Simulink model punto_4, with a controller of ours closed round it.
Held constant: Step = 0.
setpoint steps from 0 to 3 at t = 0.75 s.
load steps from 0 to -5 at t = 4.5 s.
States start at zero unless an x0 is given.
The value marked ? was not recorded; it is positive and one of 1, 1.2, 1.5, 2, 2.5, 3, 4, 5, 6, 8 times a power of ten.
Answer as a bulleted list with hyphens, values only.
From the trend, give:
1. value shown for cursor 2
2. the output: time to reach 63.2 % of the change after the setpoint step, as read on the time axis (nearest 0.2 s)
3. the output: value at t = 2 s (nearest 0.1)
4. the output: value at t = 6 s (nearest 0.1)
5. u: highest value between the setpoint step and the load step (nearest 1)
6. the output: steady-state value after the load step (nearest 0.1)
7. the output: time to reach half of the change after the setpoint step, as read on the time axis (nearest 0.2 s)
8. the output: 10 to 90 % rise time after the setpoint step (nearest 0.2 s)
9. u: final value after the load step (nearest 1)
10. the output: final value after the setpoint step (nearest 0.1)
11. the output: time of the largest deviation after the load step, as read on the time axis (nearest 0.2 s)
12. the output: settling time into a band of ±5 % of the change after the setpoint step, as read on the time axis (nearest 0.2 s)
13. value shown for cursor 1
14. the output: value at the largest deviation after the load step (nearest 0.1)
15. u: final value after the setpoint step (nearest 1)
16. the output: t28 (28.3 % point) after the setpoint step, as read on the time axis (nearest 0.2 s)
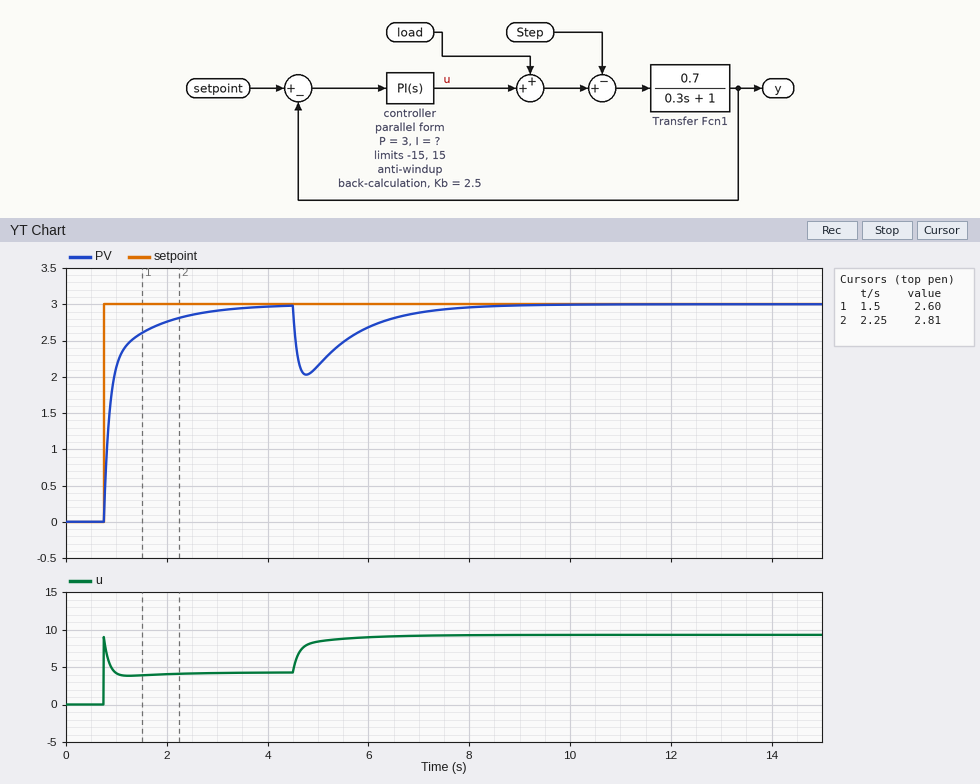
- 2.81
- 1.0 s
- 2.8
- 2.7
- 9
- 3.0
- 0.8 s
- 1.0 s
- 9
- 3.0
- 4.8 s
- 2.4 s
- 2.60
- 2.0
- 4
- 0.8 s
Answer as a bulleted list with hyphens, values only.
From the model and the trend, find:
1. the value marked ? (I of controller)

- 4
